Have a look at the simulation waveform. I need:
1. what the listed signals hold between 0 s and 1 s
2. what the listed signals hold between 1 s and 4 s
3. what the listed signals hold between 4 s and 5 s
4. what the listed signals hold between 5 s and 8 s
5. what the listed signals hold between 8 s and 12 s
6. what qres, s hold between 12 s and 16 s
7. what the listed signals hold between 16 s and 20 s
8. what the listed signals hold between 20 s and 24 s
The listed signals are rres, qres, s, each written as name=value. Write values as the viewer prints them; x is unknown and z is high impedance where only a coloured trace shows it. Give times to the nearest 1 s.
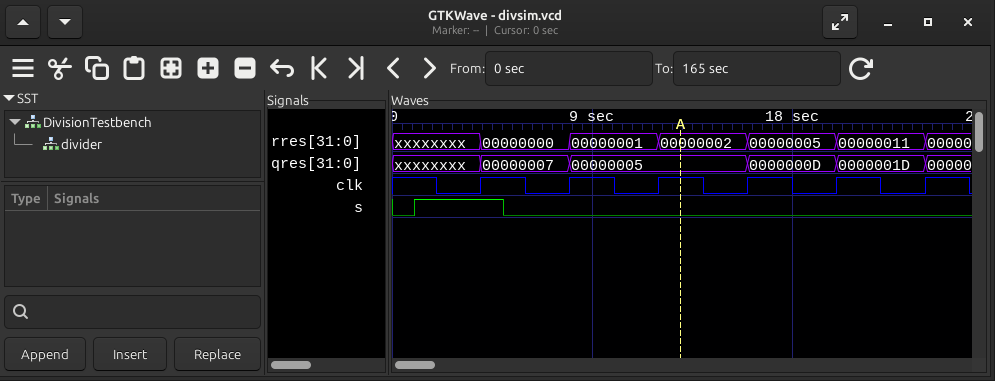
rres=xxxxxxxx, qres=xxxxxxxx, s=0
rres=xxxxxxxx, qres=xxxxxxxx, s=1
rres=00000000, qres=00000007, s=1
rres=00000000, qres=00000007, s=0
rres=00000001, qres=00000005, s=0
qres=00000005, s=0
rres=00000005, qres=0000000D, s=0
rres=00000011, qres=0000001D, s=0
